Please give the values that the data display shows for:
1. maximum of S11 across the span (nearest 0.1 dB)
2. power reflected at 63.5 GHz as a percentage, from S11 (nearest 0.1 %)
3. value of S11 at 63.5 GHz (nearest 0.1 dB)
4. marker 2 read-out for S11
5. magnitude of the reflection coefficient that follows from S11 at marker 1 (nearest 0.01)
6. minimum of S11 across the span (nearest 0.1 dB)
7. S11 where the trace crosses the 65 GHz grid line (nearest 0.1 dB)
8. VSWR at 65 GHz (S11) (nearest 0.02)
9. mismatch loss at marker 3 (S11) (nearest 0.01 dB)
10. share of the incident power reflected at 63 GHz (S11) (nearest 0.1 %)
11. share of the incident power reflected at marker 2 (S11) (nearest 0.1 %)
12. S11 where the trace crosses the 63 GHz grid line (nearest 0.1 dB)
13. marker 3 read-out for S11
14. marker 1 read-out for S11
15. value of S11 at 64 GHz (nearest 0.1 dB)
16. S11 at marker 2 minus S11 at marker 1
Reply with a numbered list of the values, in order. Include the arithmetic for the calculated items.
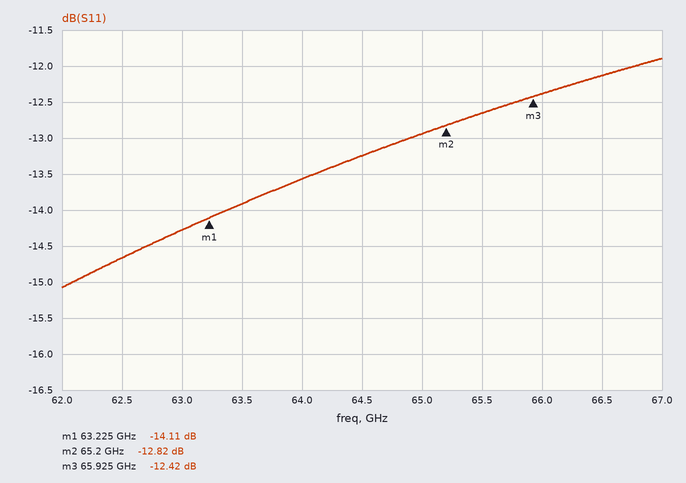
1. -11.9 dB
2. 10^(-13.9/10) ≈ 4.1 %
3. -13.9 dB
4. -12.82 dB
5. 10^(-14.11/20) ≈ 0.20
6. -15.1 dB
7. -12.9 dB
8. |Γ| = 10^(-12.9/20) = 0.2265; VSWR = (1 + 0.2265)/(1 − 0.2265) ≈ 1.59, so 1.58 to the nearest 0.02
9. −10 log10(1 − 10^(-12.42/10)) ≈ 0.26 dB
10. 10^(-14.3/10) ≈ 3.7 %
11. 10^(-12.82/10) ≈ 5.2 %
12. -14.3 dB
13. -12.42 dB
14. -14.11 dB
15. -13.6 dB
16. -12.82 − (-14.11) = 1.29 dB
